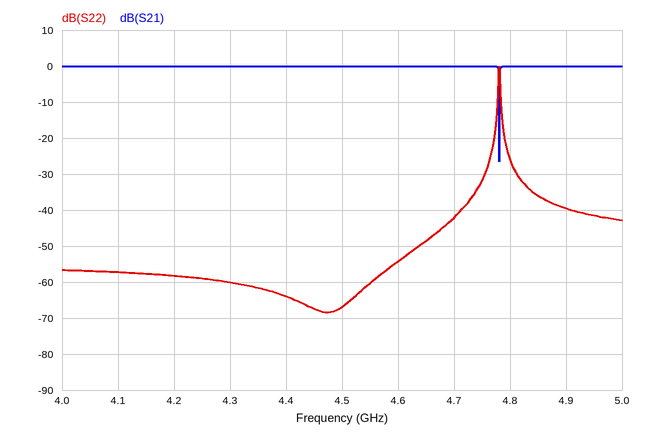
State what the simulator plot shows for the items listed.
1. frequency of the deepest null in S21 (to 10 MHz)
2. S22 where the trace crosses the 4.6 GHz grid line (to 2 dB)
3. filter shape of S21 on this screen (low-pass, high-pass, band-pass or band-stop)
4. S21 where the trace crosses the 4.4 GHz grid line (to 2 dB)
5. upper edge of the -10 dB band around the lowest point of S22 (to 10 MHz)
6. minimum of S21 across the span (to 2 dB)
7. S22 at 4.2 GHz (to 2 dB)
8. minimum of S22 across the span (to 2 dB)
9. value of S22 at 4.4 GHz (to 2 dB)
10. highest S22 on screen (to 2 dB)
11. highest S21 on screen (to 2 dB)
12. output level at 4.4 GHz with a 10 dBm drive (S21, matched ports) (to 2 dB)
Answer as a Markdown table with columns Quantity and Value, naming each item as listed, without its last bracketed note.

| Quantity | Value |
|---|---|
| frequency of the deepest null in S21 | 4.78 GHz |
| S22 where the trace crosses the 4.6 GHz grid line | -54 dB |
| filter shape of S21 on this screen | band-stop |
| S21 where the trace crosses the 4.4 GHz grid line | 0 dB |
| upper edge of the -10 dB band around the lowest point of S22 | 4.78 GHz |
| minimum of S21 across the span | -26 dB |
| S22 at 4.2 GHz | -58 dB |
| minimum of S22 across the span | -68 dB |
| value of S22 at 4.4 GHz | -64 dB |
| highest S22 on screen | 0 dB |
| highest S21 on screen | 0 dB |
| output level at 4.4 GHz with a 10 dBm drive (S21, matched ports) | 10 dBm |
